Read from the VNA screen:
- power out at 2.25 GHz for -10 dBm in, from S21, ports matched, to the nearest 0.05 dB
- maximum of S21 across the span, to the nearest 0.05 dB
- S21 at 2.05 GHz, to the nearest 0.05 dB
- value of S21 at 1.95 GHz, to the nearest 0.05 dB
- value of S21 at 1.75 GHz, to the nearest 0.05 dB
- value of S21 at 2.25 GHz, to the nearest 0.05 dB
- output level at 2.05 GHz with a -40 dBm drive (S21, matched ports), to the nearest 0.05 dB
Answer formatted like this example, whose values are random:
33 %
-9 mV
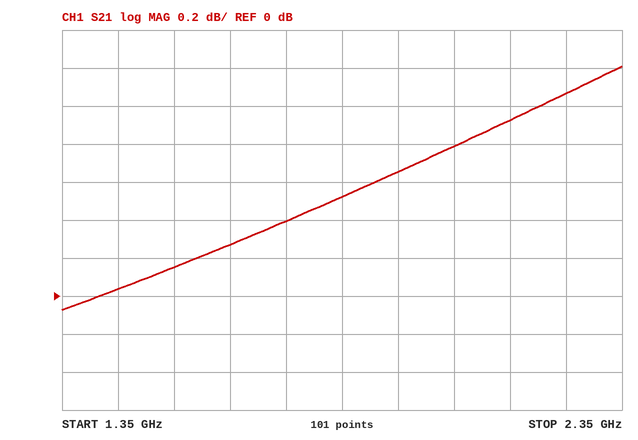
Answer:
-8.95 dBm
1.20 dB
0.80 dB
0.65 dB
0.40 dB
1.05 dB
-39.20 dBm
